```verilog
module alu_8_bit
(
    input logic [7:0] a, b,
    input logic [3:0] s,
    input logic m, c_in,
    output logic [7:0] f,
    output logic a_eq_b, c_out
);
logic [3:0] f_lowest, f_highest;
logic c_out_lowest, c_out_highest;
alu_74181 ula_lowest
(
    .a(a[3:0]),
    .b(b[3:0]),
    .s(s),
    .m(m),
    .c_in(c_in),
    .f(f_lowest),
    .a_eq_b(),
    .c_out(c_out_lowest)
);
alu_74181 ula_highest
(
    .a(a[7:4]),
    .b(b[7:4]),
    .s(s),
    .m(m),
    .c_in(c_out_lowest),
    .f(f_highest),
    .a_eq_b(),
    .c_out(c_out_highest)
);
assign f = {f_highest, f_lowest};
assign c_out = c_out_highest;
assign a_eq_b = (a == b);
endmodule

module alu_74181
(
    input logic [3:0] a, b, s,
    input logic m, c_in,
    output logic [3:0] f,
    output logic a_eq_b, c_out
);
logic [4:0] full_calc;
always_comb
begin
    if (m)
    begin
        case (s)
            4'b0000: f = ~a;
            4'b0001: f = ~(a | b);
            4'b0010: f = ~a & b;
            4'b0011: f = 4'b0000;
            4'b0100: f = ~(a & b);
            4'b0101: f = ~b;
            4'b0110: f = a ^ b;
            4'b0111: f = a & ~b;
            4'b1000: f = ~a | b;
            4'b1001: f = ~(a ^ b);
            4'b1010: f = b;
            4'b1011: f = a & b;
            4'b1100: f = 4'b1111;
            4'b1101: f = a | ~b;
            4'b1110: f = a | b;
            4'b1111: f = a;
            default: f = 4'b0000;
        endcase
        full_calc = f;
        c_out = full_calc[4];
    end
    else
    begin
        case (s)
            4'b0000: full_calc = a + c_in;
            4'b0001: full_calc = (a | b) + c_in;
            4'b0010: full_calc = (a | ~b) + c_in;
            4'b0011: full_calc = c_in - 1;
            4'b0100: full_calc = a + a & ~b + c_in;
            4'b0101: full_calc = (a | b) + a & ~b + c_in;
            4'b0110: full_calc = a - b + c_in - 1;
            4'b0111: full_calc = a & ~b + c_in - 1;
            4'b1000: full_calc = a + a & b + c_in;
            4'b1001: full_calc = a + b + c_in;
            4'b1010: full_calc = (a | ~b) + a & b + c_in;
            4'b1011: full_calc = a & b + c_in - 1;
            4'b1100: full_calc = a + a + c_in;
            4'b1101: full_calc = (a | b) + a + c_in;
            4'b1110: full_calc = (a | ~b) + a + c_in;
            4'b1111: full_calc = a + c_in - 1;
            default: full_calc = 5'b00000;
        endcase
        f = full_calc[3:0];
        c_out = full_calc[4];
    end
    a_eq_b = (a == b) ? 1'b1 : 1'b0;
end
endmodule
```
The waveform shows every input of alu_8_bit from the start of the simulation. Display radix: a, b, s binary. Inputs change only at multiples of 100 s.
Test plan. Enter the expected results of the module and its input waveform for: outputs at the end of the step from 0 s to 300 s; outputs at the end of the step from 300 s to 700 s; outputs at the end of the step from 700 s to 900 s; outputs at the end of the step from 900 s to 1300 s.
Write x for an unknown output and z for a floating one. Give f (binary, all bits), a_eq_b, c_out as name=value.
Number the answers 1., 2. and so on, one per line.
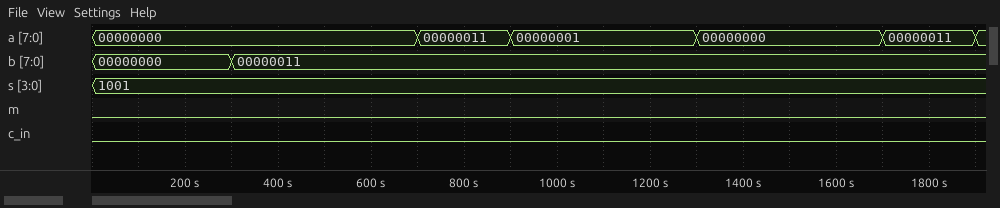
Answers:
1. f=00000000, a_eq_b=1, c_out=0
2. f=00000011, a_eq_b=0, c_out=0
3. f=00000110, a_eq_b=1, c_out=0
4. f=00000100, a_eq_b=0, c_out=0
